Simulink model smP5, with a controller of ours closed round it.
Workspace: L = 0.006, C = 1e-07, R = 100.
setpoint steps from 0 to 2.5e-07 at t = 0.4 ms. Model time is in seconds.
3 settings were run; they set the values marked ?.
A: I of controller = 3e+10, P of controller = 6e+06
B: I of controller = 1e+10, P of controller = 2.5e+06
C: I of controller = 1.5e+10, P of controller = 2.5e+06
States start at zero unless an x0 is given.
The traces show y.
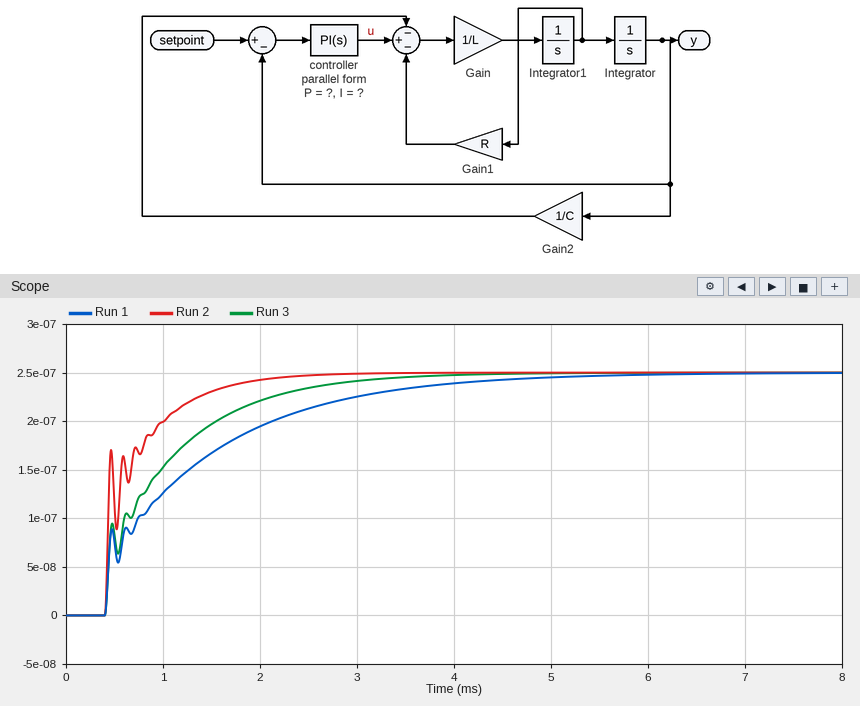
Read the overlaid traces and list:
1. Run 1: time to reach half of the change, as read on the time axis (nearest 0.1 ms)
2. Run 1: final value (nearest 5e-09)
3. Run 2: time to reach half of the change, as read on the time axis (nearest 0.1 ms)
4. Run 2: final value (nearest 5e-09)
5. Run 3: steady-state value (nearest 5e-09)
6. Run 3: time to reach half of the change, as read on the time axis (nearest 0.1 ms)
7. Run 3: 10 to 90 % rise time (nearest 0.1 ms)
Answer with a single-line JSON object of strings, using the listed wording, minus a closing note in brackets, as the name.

{"Run 1: time to reach half of the change, as read on the time axis": "1.0 ms", "Run 1: final value": "0.000000250", "Run 2: time to reach half of the change, as read on the time axis": "0.4 ms", "Run 2: final value": "0.000000250", "Run 3: steady-state value": "0.000000250", "Run 3: time to reach half of the change, as read on the time axis": "0.8 ms", "Run 3: 10 to 90 % rise time": "1.7 ms"}
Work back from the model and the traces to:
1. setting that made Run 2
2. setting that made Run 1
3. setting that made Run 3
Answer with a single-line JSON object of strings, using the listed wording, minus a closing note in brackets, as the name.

{"setting that made Run 2": "A", "setting that made Run 1": "B", "setting that made Run 3": "C"}
